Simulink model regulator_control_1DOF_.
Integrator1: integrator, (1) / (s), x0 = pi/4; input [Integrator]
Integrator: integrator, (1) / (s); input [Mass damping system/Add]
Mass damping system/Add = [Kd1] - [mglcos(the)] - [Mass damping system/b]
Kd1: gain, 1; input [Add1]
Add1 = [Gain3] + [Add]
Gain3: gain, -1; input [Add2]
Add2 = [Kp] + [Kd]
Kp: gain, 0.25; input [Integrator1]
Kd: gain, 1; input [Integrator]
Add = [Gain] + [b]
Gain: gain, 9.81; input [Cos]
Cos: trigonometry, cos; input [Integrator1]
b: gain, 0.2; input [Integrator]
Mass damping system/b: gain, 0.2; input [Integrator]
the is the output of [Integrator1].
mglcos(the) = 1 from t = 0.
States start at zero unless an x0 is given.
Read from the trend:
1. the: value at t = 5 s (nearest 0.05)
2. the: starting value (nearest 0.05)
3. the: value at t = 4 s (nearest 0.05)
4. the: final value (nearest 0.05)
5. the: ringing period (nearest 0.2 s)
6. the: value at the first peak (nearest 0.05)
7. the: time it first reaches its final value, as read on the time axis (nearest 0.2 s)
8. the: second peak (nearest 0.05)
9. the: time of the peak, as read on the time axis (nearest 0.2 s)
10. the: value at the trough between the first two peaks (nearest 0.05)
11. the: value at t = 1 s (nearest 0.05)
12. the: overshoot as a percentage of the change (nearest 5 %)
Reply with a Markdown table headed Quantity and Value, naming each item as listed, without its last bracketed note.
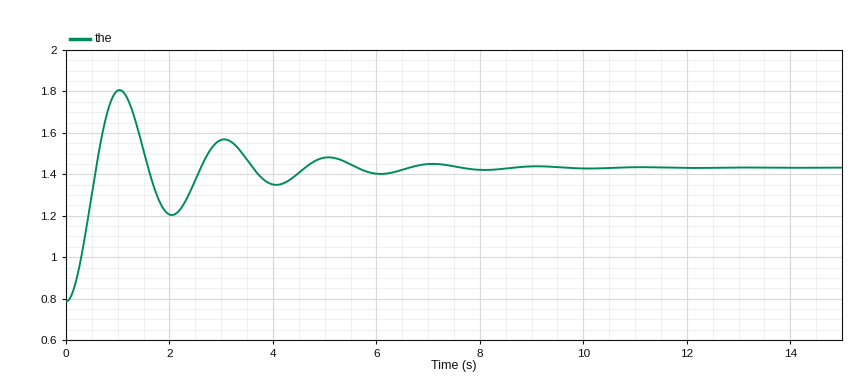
| Quantity | Value |
|---|---|
| the: value at t = 5 s | 1.50 |
| the: starting value | 0.80 |
| the: value at t = 4 s | 1.35 |
| the: final value | 1.45 |
| the: ringing period | 2.0 s |
| the: value at the first peak | 1.80 |
| the: time it first reaches its final value, as read on the time axis | 0.6 s |
| the: second peak | 1.55 |
| the: time of the peak, as read on the time axis | 1.0 s |
| the: value at the trough between the first two peaks | 1.20 |
| the: value at t = 1 s | 1.80 |
| the: overshoot as a percentage of the change | 60 % |
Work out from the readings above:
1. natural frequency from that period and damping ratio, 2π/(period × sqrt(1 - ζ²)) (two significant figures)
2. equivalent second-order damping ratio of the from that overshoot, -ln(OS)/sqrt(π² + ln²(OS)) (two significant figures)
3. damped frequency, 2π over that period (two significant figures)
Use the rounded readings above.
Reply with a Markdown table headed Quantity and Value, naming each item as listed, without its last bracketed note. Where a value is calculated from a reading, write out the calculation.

| Quantity | Value |
|---|---|
| natural frequency from that period and damping ratio, 2π/(period × sqrt(1 - ζ²)) | 2π / (2 × sqrt(1 - 0.16²)) = 3.2 rad/s |
| equivalent second-order damping ratio of the from that overshoot, -ln(OS)/sqrt(π² + ln²(OS)) | ln(0.6) = -0.511; 0.511 / sqrt(9.870 + 0.261) = 0.16 |
| damped frequency, 2π over that period | 2π / 2 = 3.1 rad/s |
